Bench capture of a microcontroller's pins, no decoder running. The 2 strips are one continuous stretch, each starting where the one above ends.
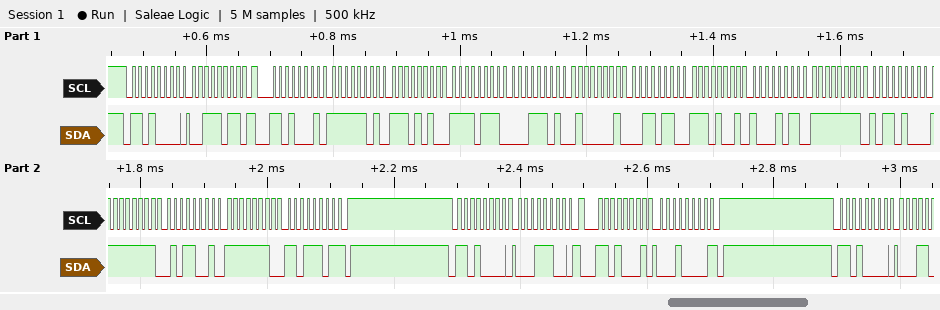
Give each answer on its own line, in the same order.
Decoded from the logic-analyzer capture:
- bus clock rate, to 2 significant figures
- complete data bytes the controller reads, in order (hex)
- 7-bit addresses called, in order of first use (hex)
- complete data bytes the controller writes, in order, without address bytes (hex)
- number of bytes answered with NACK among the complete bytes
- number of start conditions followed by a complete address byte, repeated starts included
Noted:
100 kHz
FD EA F7 1D 41 36 E9 8B FF B4 FF 59 FE DD 10
0x68
3B 1C
2
5
